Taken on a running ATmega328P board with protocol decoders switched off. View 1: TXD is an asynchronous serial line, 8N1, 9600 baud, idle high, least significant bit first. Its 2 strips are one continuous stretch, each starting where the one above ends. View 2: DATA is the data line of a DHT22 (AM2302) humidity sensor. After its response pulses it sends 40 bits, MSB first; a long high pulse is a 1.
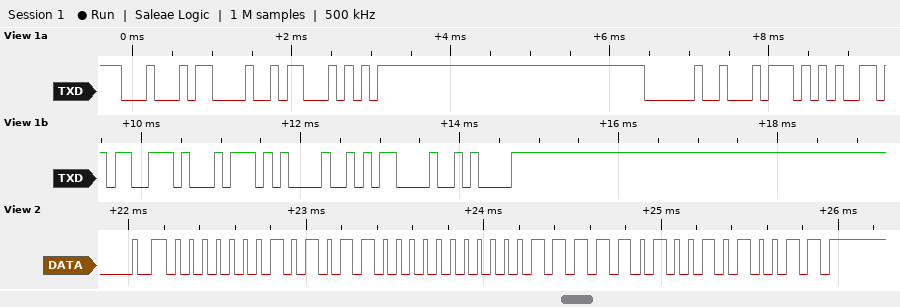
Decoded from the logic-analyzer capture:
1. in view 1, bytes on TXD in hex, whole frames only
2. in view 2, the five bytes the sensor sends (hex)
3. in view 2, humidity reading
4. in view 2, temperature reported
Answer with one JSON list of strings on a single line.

["44 48 54 20 74 65 73 74 21 0D 0A", "01 58 00 FA 53", "34.4 %", "25.0 °C"]
